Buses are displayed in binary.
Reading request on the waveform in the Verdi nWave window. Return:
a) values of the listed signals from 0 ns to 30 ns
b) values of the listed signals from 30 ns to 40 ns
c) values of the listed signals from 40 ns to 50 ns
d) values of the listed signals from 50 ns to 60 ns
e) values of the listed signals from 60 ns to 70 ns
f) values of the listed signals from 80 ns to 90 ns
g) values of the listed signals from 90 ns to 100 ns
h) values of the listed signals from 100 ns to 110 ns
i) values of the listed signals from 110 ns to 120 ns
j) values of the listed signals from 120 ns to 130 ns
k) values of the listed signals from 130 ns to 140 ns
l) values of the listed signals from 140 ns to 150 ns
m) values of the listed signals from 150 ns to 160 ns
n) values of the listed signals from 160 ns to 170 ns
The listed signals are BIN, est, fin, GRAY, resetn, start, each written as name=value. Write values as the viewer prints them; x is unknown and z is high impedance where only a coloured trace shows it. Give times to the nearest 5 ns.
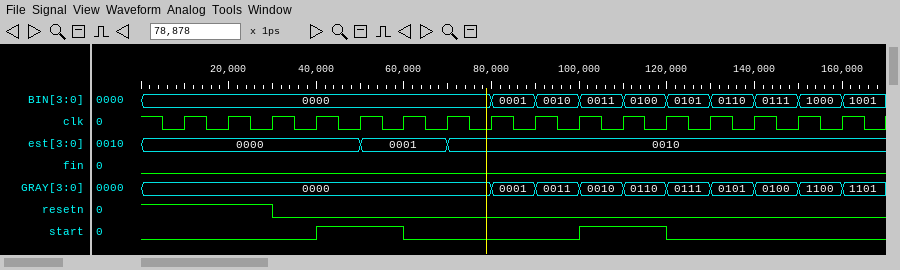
BIN=0000, est=0000, fin=0, GRAY=0000, resetn=1, start=0
BIN=0000, est=0000, fin=0, GRAY=0000, resetn=0, start=0
BIN=0000, est=0000, fin=0, GRAY=0000, resetn=0, start=1
BIN=0000, est=0001, fin=0, GRAY=0000, resetn=0, start=1
BIN=0000, est=0001, fin=0, GRAY=0000, resetn=0, start=0
BIN=0001, est=0010, fin=0, GRAY=0001, resetn=0, start=0
BIN=0010, est=0010, fin=0, GRAY=0011, resetn=0, start=0
BIN=0011, est=0010, fin=0, GRAY=0010, resetn=0, start=1
BIN=0100, est=0010, fin=0, GRAY=0110, resetn=0, start=1
BIN=0101, est=0010, fin=0, GRAY=0111, resetn=0, start=0
BIN=0110, est=0010, fin=0, GRAY=0101, resetn=0, start=0
BIN=0111, est=0010, fin=0, GRAY=0100, resetn=0, start=0
BIN=1000, est=0010, fin=0, GRAY=1100, resetn=0, start=0
BIN=1001, est=0010, fin=0, GRAY=1101, resetn=0, start=0
